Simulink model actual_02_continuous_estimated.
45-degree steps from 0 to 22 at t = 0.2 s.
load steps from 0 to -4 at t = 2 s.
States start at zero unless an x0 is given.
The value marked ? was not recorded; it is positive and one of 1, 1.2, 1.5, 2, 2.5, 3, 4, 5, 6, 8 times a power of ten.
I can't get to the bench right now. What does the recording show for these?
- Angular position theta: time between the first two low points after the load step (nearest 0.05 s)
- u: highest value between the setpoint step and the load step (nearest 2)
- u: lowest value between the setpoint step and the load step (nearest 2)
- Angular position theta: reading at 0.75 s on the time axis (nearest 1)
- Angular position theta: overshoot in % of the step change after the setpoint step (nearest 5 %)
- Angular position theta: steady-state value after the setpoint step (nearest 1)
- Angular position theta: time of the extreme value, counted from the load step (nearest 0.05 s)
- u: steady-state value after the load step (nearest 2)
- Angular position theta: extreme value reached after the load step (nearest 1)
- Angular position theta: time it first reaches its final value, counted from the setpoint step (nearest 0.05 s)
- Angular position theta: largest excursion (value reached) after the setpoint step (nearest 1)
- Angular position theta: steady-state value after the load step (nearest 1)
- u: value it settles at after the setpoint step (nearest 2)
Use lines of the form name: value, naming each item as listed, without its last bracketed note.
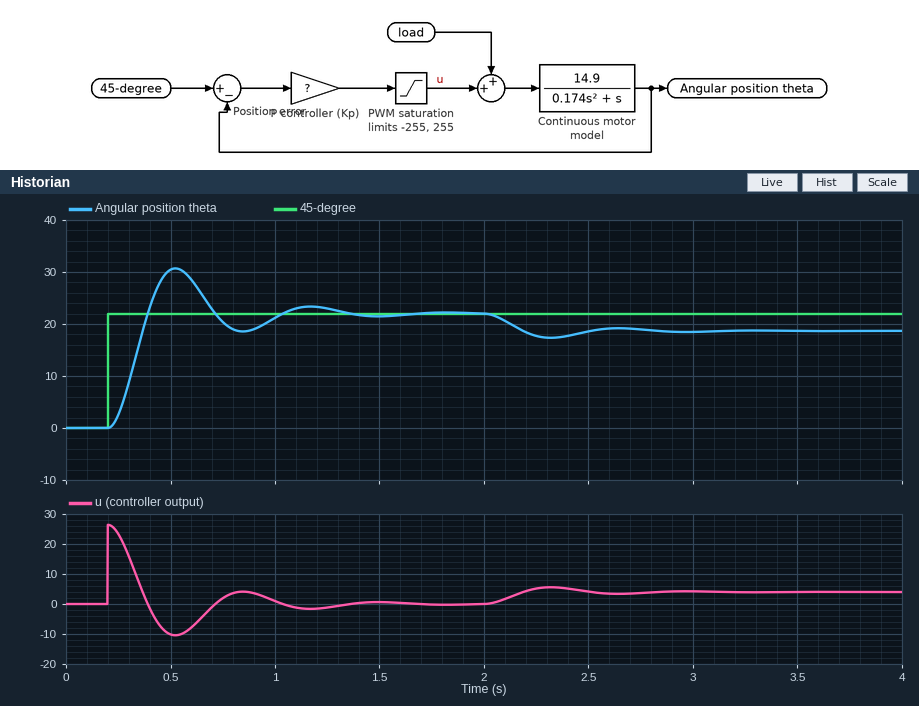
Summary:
Angular position theta: time between the first two low points after the load step: 0.65 s
u: highest value between the setpoint step and the load step: 26
u: lowest value between the setpoint step and the load step: -10
Angular position theta: reading at 0.75 s on the time axis: 20
Angular position theta: overshoot in % of the step change after the setpoint step: 40 %
Angular position theta: steady-state value after the setpoint step: 22
Angular position theta: time of the extreme value, counted from the load step: 0.30 s
u: steady-state value after the load step: 4
Angular position theta: extreme value reached after the load step: 17
Angular position theta: time it first reaches its final value, counted from the setpoint step: 0.20 s
Angular position theta: largest excursion (value reached) after the setpoint step: 31
Angular position theta: steady-state value after the load step: 19
u: value it settles at after the setpoint step: 0
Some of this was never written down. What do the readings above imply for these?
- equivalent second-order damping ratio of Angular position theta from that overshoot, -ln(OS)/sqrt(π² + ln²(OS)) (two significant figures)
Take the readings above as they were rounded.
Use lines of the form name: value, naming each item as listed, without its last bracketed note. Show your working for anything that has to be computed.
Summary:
equivalent second-order damping ratio of Angular position theta from that overshoot, -ln(OS)/sqrt(π² + ln²(OS)): ln(0.4) = -0.916; 0.916 / sqrt(9.870 + 0.840) = 0.28
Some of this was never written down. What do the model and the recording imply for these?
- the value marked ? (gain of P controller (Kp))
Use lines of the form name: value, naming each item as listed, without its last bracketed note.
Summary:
the value marked ? (gain of P controller (Kp)): 1.2
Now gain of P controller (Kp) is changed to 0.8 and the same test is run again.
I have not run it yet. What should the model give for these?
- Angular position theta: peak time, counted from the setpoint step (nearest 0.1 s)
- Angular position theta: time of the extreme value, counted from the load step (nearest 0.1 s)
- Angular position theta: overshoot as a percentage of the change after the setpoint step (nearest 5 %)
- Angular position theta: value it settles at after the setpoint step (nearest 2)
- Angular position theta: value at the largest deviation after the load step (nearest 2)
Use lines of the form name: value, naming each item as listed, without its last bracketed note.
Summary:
Angular position theta: peak time, counted from the setpoint step: 0.4 s
Angular position theta: time of the extreme value, counted from the load step: 0.4 s
Angular position theta: overshoot as a percentage of the change after the setpoint step: 30 %
Angular position theta: value it settles at after the setpoint step: 22
Angular position theta: value at the largest deviation after the load step: 16
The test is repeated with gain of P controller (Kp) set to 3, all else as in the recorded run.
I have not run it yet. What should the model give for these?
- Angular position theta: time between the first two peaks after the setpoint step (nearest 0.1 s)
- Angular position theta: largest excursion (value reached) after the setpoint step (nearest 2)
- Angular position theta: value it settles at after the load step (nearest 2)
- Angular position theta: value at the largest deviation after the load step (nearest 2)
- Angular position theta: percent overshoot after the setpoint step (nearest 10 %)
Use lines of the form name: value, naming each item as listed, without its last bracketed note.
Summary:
Angular position theta: time between the first two peaks after the setpoint step: 0.4 s
Angular position theta: largest excursion (value reached) after the setpoint step: 34
Angular position theta: value it settles at after the load step: 20
Angular position theta: value at the largest deviation after the load step: 20
Angular position theta: percent overshoot after the setpoint step: 60 %
